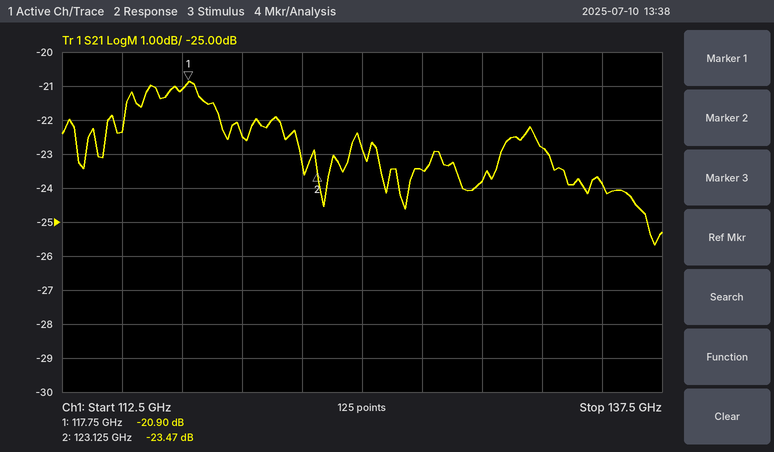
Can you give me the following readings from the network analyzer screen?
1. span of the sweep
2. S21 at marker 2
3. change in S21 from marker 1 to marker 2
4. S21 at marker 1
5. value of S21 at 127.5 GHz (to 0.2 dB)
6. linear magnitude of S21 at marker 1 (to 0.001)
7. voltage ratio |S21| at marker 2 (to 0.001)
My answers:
25 GHz
-23.47 dB
-2.57 dB
-20.90 dB
-23.4 dB
0.090
0.067
